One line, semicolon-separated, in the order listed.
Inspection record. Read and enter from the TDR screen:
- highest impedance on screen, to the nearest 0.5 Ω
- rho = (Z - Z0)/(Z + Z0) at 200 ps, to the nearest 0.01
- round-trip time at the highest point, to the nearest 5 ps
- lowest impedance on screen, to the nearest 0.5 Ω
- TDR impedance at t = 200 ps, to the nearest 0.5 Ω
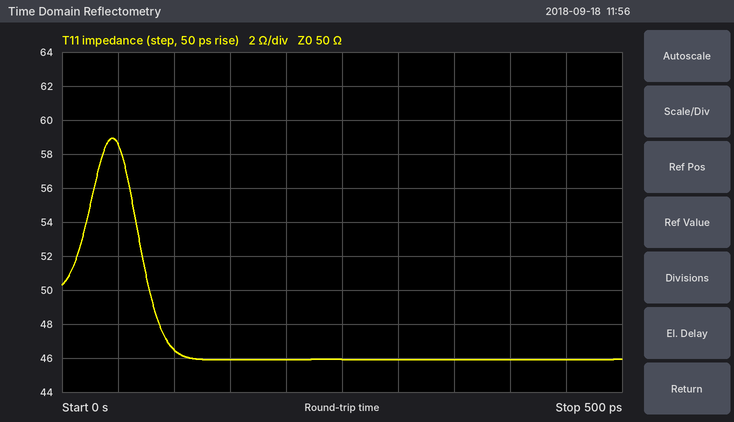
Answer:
59.0 Ω; -0.04; 45 ps; 46.0 Ω; 46.0 Ω
